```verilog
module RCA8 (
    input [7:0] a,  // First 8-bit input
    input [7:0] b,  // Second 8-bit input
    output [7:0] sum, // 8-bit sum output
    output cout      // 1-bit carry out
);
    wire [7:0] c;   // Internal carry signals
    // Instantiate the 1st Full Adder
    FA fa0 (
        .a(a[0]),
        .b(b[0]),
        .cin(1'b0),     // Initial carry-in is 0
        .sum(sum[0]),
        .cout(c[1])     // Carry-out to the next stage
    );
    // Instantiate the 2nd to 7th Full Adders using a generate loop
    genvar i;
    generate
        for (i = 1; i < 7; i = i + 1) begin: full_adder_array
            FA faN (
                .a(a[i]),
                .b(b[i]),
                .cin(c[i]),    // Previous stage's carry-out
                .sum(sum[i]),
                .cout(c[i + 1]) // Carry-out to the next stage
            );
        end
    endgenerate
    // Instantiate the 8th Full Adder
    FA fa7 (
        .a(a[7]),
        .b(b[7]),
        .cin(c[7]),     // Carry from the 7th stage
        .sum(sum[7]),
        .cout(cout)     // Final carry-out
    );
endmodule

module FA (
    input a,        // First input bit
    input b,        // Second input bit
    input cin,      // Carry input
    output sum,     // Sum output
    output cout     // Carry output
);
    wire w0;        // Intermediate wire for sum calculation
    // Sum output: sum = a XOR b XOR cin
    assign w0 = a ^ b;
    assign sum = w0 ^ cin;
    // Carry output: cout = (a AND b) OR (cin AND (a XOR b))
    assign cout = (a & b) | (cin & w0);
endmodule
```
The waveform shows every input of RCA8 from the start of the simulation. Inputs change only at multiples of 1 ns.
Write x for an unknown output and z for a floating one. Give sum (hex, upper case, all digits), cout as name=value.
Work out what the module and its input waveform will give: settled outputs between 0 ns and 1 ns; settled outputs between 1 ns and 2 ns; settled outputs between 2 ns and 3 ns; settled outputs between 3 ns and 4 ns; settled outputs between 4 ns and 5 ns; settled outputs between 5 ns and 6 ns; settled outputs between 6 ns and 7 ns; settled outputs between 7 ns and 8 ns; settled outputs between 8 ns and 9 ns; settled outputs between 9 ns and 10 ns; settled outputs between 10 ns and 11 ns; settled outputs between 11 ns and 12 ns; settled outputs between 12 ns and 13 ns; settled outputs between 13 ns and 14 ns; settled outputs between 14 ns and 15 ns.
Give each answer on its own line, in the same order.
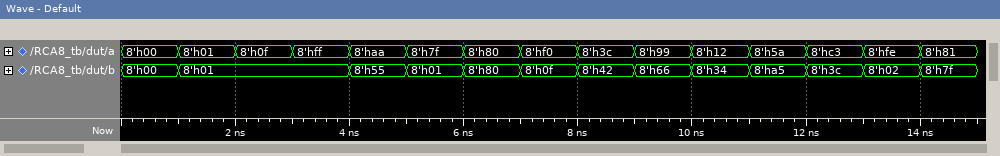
sum=00, cout=0
sum=02, cout=0
sum=10, cout=0
sum=00, cout=1
sum=FF, cout=0
sum=80, cout=0
sum=00, cout=1
sum=FF, cout=0
sum=7E, cout=0
sum=FF, cout=0
sum=46, cout=0
sum=FF, cout=0
sum=FF, cout=0
sum=00, cout=1
sum=00, cout=1
